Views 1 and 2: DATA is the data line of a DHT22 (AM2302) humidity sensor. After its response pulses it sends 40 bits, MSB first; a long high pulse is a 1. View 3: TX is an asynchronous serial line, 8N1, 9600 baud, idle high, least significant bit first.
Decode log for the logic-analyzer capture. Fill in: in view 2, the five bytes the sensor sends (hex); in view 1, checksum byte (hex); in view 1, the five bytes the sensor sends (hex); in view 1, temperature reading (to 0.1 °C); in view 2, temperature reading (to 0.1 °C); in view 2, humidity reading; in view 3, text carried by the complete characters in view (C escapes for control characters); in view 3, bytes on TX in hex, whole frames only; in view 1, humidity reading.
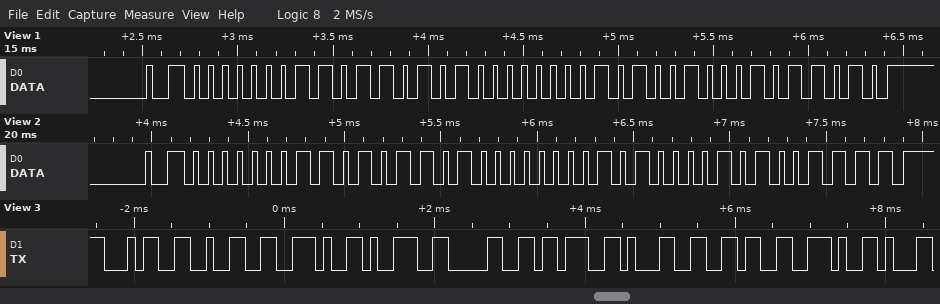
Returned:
01 AD 00 A1 4F
0x5A
01 B5 00 A4 5A
16.4 °C
16.1 °C
42.9 %
"42.90;16."
34 32 2E 39 30 3B 31 36 2E
43.7 %
